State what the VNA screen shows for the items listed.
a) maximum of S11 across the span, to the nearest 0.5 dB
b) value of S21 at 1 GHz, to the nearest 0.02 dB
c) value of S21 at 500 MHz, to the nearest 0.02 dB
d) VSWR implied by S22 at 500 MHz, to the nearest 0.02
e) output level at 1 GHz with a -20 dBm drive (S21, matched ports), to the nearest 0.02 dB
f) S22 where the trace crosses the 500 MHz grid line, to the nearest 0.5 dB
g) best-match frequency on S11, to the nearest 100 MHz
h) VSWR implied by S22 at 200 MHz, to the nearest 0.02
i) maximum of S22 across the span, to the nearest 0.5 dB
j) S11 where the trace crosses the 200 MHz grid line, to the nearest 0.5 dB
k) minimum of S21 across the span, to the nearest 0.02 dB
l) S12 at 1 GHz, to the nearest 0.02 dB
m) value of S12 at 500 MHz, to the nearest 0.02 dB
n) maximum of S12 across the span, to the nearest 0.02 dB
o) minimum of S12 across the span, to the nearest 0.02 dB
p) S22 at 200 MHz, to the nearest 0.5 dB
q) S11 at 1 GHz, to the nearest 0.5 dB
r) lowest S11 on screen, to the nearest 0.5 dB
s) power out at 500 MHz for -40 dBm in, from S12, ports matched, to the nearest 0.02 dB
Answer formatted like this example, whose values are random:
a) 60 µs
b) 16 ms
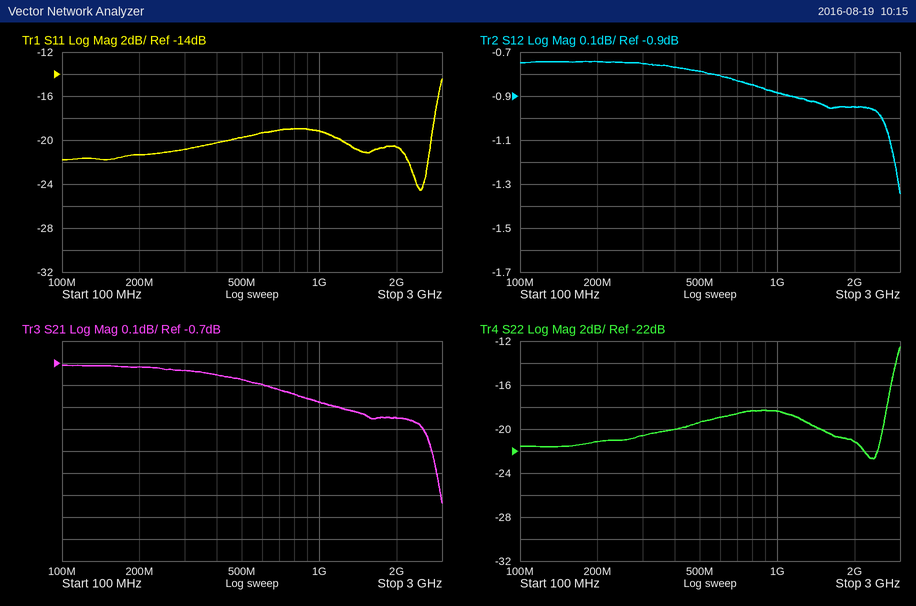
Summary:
a) -14.5 dB
b) -0.88 dB
c) -0.78 dB
d) 1.24
e) -20.88 dBm
f) -19.5 dB
g) 2.5 GHz
h) 1.20
i) -12.5 dB
j) -21.5 dB
k) -1.34 dB
l) -0.88 dB
m) -0.78 dB
n) -0.74 dB
o) -1.34 dB
p) -21.0 dB
q) -19.0 dB
r) -24.5 dB
s) -40.78 dBm
